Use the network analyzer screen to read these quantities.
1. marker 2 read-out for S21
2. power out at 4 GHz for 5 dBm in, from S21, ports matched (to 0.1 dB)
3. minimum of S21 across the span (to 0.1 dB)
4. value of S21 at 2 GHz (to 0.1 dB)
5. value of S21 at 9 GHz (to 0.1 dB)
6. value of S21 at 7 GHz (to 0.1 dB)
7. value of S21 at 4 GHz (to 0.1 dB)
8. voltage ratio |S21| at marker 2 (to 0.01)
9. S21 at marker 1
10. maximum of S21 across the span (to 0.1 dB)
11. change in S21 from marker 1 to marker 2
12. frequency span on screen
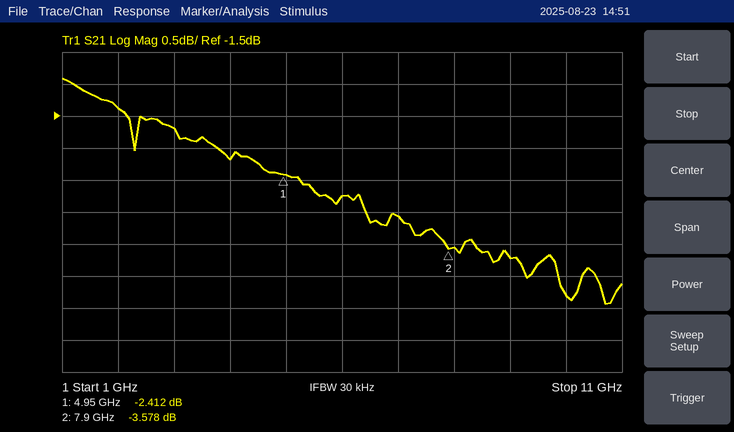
-3.578 dB
2.8 dBm
-4.4 dB
-1.4 dB
-3.7 dB
-3.1 dB
-2.2 dB
0.66
-2.412 dB
-0.9 dB
-1.166 dB
10 GHz
